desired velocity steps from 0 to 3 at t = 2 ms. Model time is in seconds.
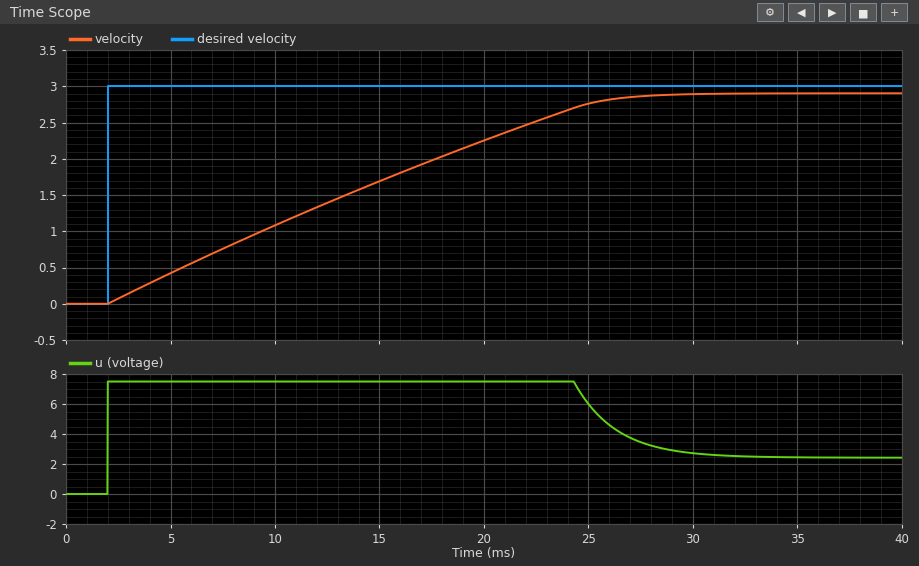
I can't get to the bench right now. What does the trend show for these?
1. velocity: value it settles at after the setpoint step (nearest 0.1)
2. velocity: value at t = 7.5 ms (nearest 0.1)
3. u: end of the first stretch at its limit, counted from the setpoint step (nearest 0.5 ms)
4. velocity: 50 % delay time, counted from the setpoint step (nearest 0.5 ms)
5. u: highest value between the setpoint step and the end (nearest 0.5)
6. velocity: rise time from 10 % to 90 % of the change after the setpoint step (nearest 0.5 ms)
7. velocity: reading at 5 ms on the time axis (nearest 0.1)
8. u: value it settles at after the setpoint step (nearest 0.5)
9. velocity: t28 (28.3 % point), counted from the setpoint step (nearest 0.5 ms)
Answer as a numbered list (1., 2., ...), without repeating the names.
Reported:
1. 2.9
2. 0.8
3. 22.5 ms
4. 11.0 ms
5. 7.5
6. 19.5 ms
7. 0.4
8. 2.5
9. 6.0 ms
